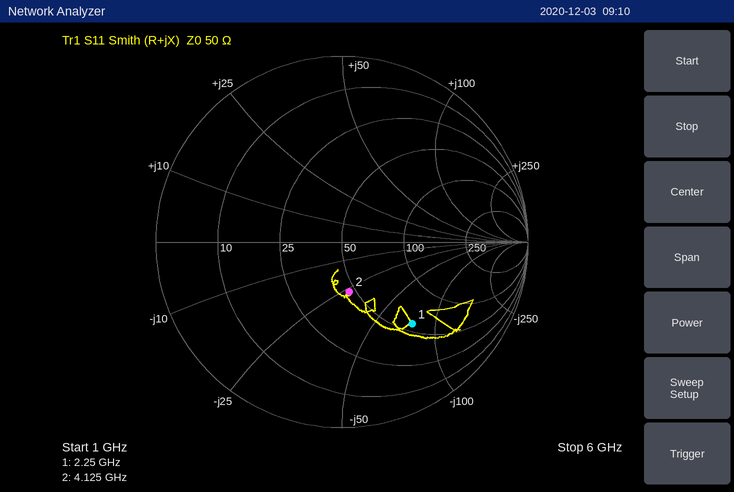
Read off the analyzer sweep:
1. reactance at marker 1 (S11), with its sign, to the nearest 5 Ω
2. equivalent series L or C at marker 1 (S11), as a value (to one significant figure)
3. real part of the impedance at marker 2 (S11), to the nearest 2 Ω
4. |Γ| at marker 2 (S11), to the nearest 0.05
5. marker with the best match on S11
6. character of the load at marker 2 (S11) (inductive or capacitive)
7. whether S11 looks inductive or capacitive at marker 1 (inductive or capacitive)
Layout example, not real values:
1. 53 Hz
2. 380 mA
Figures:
1. -75 Ω
2. 900 fF
3. 46 Ω
4. 0.25
5. marker 2
6. capacitive
7. capacitive
